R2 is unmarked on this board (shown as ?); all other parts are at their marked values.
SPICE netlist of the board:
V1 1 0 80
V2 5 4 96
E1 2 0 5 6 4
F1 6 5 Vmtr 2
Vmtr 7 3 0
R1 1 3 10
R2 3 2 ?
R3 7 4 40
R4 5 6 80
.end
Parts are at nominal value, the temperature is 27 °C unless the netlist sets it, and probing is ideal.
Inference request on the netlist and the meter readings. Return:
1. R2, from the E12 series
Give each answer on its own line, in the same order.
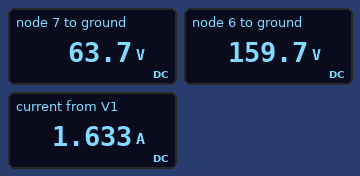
39 Ω
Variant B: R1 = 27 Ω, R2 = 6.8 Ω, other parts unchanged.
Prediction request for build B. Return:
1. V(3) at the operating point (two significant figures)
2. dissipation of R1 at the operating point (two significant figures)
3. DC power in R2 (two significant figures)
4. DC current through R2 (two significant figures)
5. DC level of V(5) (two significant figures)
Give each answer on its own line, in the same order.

16 V
150 W
38 W
2.4 A
110 V
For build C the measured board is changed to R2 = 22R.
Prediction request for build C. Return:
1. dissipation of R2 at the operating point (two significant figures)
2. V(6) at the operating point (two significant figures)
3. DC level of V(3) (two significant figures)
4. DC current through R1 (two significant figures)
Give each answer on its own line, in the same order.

140 W
150 V
55 V
2.5 A
